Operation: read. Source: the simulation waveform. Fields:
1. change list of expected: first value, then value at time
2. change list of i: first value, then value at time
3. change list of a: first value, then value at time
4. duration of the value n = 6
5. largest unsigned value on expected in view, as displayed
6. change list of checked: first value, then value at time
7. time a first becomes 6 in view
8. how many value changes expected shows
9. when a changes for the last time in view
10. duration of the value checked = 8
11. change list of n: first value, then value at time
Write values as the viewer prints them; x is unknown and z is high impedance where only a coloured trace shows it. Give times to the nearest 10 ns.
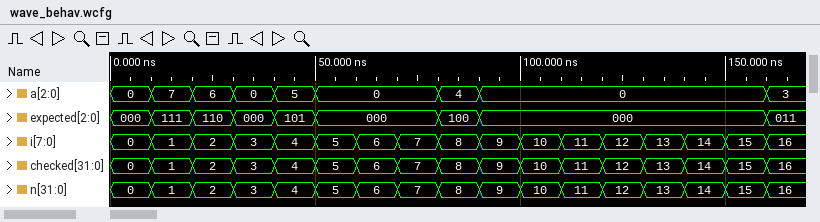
000, 111 at 10 ns, 110 at 20 ns, 000 at 30 ns, 101 at 40 ns, 000 at 50 ns, 100 at 80 ns, 000 at 90 ns, 011 at 160 ns
0, 1 at 10 ns, 2 at 20 ns, 3 at 30 ns, 4 at 40 ns, 5 at 50 ns, 6 at 60 ns, 7 at 70 ns, 8 at 80 ns, 9 at 90 ns, 10 at 100 ns, 11 at 110 ns, 12 at 120 ns, 13 at 130 ns, 14 at 140 ns, 15 at 150 ns, 16 at 160 ns
0, 7 at 10 ns, 6 at 20 ns, 0 at 30 ns, 5 at 40 ns, 0 at 50 ns, 4 at 80 ns, 0 at 90 ns, 3 at 160 ns
10 ns
111
0, 1 at 10 ns, 2 at 20 ns, 3 at 30 ns, 4 at 40 ns, 5 at 50 ns, 6 at 60 ns, 7 at 70 ns, 8 at 80 ns, 9 at 90 ns, 10 at 100 ns, 11 at 110 ns, 12 at 120 ns, 13 at 130 ns, 14 at 140 ns, 15 at 150 ns, 16 at 160 ns
20 ns
8
160 ns
10 ns
0, 1 at 10 ns, 2 at 20 ns, 3 at 30 ns, 4 at 40 ns, 5 at 50 ns, 6 at 60 ns, 7 at 70 ns, 8 at 80 ns, 9 at 90 ns, 10 at 100 ns, 11 at 110 ns, 12 at 120 ns, 13 at 130 ns, 14 at 140 ns, 15 at 150 ns, 16 at 160 ns
